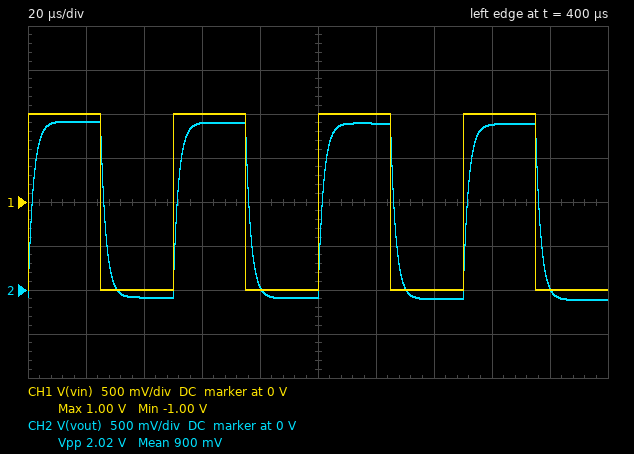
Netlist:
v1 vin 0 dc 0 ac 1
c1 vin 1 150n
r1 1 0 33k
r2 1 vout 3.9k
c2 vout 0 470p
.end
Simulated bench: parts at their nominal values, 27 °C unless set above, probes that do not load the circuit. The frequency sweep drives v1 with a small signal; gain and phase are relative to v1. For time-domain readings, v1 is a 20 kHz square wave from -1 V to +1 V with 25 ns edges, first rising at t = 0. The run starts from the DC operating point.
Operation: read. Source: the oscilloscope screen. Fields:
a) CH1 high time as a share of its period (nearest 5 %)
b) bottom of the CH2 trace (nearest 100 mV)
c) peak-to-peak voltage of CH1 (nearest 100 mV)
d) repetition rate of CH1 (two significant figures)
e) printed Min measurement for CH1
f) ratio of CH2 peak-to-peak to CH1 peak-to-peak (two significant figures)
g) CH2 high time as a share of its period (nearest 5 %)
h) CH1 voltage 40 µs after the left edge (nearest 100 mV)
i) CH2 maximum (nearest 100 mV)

50 %
-100 mV
2.0 V
20 kHz
-1.00 V
1.0
50 %
-1.0 V
1.9 V
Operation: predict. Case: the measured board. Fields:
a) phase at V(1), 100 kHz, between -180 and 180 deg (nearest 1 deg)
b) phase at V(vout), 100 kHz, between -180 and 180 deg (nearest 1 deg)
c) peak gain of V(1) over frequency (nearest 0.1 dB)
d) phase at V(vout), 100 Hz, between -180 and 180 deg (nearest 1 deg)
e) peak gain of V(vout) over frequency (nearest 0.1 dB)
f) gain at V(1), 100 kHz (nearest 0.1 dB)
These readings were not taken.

0 deg
-49 deg
0 dB
18 deg
0 dB
0 dB
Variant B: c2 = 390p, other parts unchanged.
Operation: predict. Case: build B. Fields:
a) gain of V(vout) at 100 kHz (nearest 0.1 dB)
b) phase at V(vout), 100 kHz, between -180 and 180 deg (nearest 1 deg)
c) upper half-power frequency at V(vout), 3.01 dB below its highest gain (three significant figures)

-2.8 dB
-44 deg
105 kHz
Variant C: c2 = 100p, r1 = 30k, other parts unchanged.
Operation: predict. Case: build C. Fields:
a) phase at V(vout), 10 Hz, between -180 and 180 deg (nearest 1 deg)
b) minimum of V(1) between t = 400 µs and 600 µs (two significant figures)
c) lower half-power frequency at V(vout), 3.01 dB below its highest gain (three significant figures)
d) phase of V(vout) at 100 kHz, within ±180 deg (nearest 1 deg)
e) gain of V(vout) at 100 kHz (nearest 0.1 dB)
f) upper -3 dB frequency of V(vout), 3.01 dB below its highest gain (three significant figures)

74 deg
-130 mV
35.3 Hz
-14 deg
-0.3 dB
408 kHz
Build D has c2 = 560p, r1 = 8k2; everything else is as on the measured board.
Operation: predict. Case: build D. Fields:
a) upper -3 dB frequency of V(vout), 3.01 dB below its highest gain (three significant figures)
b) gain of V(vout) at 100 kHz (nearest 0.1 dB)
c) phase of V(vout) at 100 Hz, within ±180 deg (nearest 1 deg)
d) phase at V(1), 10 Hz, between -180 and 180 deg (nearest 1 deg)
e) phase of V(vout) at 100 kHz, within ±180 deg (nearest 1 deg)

73.4 kHz
-4.6 dB
52 deg
86 deg
-54 deg
